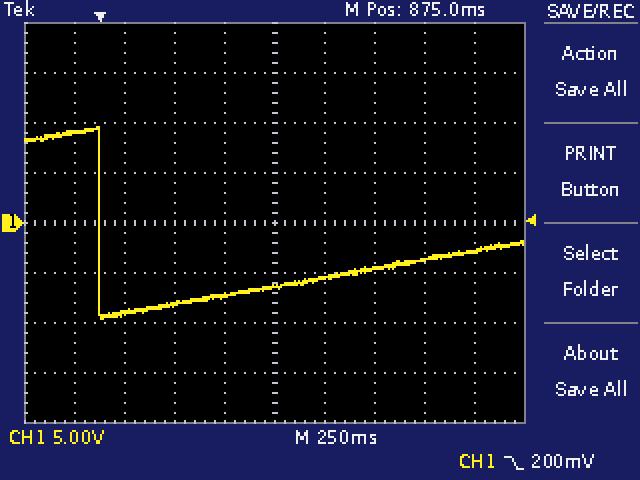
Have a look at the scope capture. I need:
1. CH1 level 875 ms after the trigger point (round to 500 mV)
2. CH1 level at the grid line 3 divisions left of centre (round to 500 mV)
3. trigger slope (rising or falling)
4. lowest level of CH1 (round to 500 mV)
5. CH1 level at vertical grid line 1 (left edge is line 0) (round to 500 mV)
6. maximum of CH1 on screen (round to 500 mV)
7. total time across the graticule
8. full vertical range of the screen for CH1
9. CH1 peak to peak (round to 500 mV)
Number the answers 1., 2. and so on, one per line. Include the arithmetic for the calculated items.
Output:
1. -6.5 V
2. -9.0 V
3. falling
4. -9.5 V
5. 9.0 V
6. 9.5 V
7. 2.5 s
8. 40 V
9. 9.5 V − (-9.5 V) = 19.0 V
